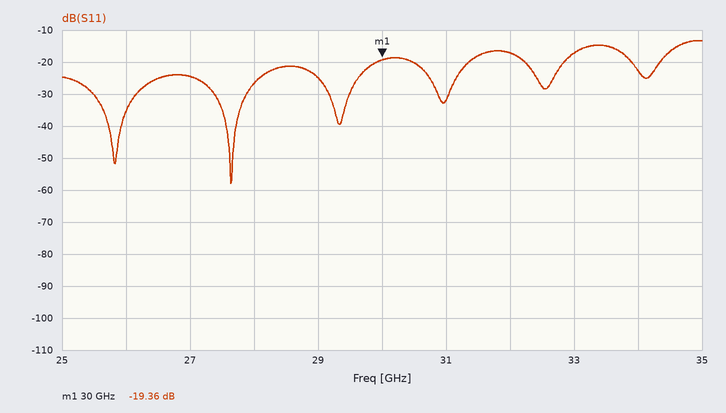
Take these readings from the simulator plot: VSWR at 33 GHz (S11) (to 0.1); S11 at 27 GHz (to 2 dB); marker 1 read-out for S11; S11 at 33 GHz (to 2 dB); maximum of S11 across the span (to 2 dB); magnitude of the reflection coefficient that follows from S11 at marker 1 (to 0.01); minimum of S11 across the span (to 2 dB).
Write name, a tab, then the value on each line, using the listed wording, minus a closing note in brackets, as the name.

VSWR at 33 GHz (S11)	1.3
S11 at 27 GHz	-24 dB
marker 1 read-out for S11	-19.36 dB
S11 at 33 GHz	-18 dB
maximum of S11 across the span	-14 dB
magnitude of the reflection coefficient that follows from S11 at marker 1	0.11
minimum of S11 across the span	-58 dB
